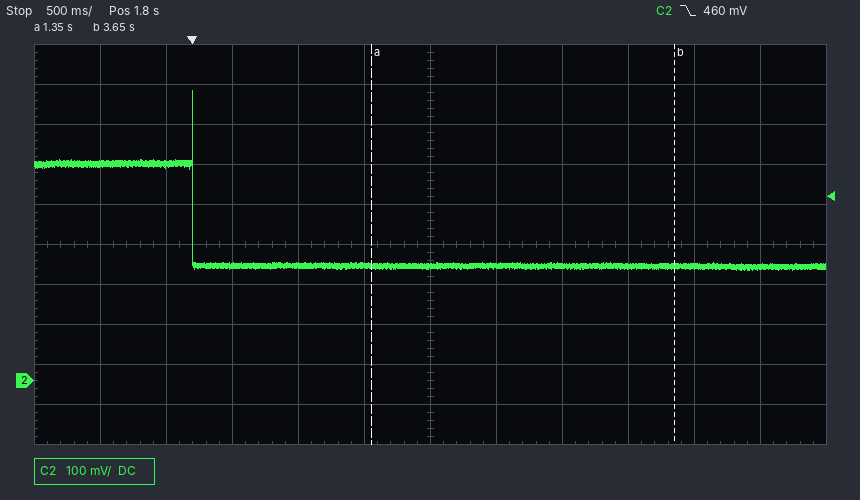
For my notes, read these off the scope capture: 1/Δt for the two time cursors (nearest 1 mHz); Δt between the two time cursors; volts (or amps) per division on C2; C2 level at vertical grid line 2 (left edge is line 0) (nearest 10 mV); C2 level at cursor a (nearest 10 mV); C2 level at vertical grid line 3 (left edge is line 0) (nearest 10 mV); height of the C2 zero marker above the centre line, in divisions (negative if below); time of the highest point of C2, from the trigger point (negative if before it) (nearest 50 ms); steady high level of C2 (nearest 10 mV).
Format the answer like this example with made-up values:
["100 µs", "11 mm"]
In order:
["435 mHz", "2.30 s", "100 mV", "540 mV", "290 mV", "290 mV", "-3.4 div", "0 ms", "540 mV"]
